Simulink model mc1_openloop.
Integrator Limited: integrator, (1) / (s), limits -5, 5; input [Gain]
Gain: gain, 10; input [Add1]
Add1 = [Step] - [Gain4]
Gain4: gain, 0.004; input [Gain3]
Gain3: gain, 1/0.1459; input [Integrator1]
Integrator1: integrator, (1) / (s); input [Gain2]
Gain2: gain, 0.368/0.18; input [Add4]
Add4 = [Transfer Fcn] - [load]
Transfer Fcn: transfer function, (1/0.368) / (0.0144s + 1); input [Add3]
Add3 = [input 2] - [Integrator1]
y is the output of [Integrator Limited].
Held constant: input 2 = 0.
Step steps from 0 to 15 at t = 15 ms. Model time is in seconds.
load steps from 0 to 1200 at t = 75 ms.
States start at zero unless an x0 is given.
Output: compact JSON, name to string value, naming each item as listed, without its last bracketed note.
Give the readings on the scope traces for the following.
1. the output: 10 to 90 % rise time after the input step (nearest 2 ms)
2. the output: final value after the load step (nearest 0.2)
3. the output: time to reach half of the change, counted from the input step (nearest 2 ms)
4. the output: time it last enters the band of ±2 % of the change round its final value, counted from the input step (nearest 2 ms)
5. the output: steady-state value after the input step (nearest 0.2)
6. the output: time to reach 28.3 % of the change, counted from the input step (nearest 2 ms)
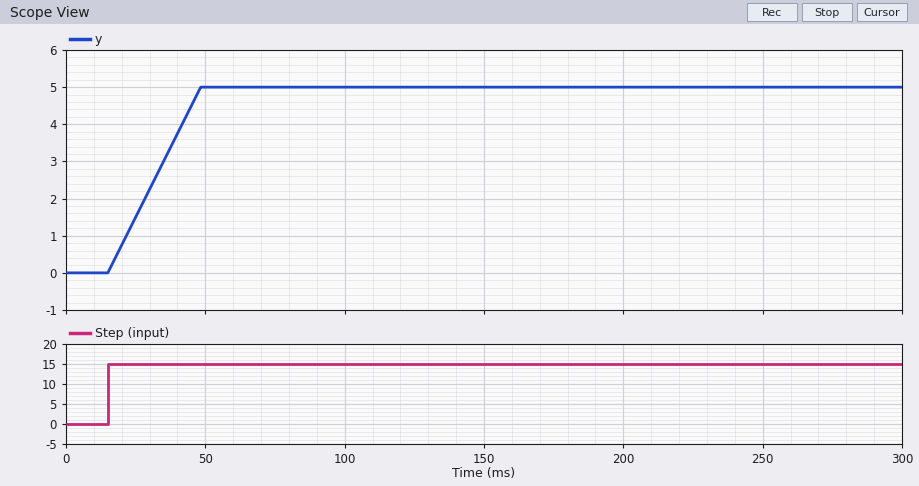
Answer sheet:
{"the output: 10 to 90 % rise time after the input step": "26 ms", "the output: final value after the load step": "5.0", "the output: time to reach half of the change, counted from the input step": "16 ms", "the output: time it last enters the band of ±2 % of the change round its final value, counted from the input step": "32 ms", "the output: steady-state value after the input step": "5.0", "the output: time to reach 28.3 % of the change, counted from the input step": "10 ms"}
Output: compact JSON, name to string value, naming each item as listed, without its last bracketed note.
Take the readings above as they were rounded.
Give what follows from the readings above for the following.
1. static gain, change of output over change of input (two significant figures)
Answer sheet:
{"static gain, change of output over change of input": "0.33"}
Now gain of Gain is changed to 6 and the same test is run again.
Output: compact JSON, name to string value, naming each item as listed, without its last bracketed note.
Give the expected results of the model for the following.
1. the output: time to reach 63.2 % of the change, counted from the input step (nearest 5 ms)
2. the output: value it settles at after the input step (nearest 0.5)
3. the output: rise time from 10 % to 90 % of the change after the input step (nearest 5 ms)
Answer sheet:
{"the output: time to reach 63.2 % of the change, counted from the input step": "35 ms", "the output: value it settles at after the input step": "5.0", "the output: rise time from 10 % to 90 % of the change after the input step": "45 ms"}
